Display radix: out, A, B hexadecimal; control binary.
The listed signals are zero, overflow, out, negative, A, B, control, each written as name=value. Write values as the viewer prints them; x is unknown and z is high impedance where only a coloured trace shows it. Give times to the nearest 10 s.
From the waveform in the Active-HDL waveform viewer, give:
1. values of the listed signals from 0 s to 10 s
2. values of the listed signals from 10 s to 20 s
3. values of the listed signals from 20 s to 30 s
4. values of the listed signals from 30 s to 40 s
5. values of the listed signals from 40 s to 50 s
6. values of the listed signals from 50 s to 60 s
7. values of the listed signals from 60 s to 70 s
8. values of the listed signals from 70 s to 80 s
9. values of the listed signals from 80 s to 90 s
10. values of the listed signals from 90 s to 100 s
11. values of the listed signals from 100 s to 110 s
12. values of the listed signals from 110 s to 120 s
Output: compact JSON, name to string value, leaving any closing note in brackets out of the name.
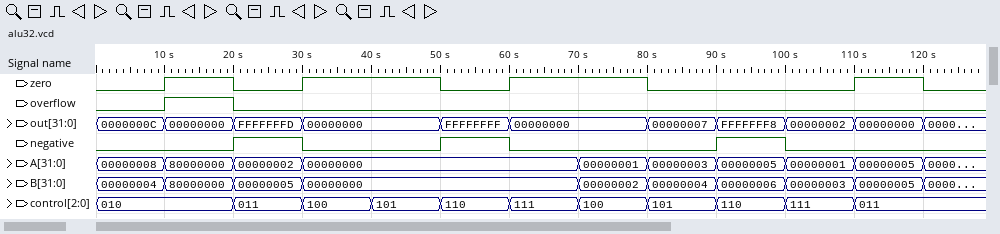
{"values of the listed signals from 0 s to 10 s": "zero=0, overflow=0, out=0000000C, negative=0, A=00000008, B=00000004, control=010", "values of the listed signals from 10 s to 20 s": "zero=1, overflow=1, out=00000000, negative=0, A=80000000, B=80000000, control=010", "values of the listed signals from 20 s to 30 s": "zero=0, overflow=0, out=FFFFFFFD, negative=1, A=00000002, B=00000005, control=011", "values of the listed signals from 30 s to 40 s": "zero=1, overflow=0, out=00000000, negative=0, A=00000000, B=00000000, control=100", "values of the listed signals from 40 s to 50 s": "zero=1, overflow=0, out=00000000, negative=0, A=00000000, B=00000000, control=101", "values of the listed signals from 50 s to 60 s": "zero=0, overflow=0, out=FFFFFFFF, negative=1, A=00000000, B=00000000, control=110", "values of the listed signals from 60 s to 70 s": "zero=1, overflow=0, out=00000000, negative=0, A=00000000, B=00000000, control=111", "values of the listed signals from 70 s to 80 s": "zero=1, overflow=0, out=00000000, negative=0, A=00000001, B=00000002, control=100", "values of the listed signals from 80 s to 90 s": "zero=0, overflow=0, out=00000007, negative=0, A=00000003, B=00000004, control=101", "values of the listed signals from 90 s to 100 s": "zero=0, overflow=0, out=FFFFFFF8, negative=1, A=00000005, B=00000006, control=110", "values of the listed signals from 100 s to 110 s": "zero=0, overflow=0, out=00000002, negative=0, A=00000001, B=00000003, control=111", "values of the listed signals from 110 s to 120 s": "zero=1, overflow=0, out=00000000, negative=0, A=00000005, B=00000005, control=011"}
